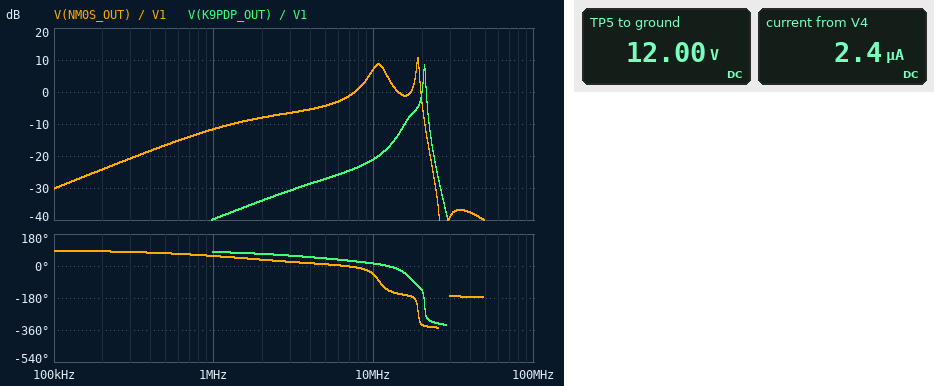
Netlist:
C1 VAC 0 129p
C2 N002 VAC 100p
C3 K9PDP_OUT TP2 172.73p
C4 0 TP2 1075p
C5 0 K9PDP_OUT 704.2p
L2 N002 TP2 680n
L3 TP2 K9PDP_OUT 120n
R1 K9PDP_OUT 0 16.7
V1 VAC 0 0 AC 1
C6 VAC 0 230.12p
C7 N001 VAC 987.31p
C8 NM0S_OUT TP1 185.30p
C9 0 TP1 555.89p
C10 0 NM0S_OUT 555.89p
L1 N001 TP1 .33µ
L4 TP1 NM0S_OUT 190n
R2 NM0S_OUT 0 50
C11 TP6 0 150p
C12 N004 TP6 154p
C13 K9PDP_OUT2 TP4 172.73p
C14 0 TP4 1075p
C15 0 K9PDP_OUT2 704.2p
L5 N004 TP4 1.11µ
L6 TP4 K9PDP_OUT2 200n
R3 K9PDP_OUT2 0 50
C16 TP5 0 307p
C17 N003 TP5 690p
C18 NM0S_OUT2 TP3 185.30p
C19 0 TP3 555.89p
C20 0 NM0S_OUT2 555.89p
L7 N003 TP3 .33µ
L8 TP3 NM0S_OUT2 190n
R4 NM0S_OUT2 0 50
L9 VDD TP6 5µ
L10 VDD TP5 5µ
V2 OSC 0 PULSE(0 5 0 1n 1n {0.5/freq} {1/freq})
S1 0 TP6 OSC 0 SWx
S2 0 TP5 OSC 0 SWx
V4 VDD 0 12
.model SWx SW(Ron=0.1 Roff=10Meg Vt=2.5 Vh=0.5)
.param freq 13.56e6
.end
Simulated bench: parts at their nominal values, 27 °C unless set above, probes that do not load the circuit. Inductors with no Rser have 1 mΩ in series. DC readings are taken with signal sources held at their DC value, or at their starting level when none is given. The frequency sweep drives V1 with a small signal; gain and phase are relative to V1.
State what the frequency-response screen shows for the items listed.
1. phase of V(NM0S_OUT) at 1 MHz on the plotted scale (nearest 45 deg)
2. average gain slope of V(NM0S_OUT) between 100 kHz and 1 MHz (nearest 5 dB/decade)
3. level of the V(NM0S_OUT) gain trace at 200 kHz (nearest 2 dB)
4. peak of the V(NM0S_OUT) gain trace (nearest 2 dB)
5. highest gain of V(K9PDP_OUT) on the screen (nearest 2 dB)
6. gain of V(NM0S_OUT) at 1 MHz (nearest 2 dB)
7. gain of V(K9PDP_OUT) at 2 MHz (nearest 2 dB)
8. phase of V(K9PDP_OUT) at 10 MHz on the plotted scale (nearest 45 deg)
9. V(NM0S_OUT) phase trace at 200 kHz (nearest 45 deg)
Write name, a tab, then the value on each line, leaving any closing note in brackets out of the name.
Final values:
phase of V(NM0S_OUT) at 1 MHz on the plotted scale	45 deg
average gain slope of V(NM0S_OUT) between 100 kHz and 1 MHz	20 dB/decade
level of the V(NM0S_OUT) gain trace at 200 kHz	-24 dB
peak of the V(NM0S_OUT) gain trace	10 dB
highest gain of V(K9PDP_OUT) on the screen	8 dB
gain of V(NM0S_OUT) at 1 MHz	-12 dB
gain of V(K9PDP_OUT) at 2 MHz	-34 dB
phase of V(K9PDP_OUT) at 10 MHz on the plotted scale	0 deg
V(NM0S_OUT) phase trace at 200 kHz	90 deg
